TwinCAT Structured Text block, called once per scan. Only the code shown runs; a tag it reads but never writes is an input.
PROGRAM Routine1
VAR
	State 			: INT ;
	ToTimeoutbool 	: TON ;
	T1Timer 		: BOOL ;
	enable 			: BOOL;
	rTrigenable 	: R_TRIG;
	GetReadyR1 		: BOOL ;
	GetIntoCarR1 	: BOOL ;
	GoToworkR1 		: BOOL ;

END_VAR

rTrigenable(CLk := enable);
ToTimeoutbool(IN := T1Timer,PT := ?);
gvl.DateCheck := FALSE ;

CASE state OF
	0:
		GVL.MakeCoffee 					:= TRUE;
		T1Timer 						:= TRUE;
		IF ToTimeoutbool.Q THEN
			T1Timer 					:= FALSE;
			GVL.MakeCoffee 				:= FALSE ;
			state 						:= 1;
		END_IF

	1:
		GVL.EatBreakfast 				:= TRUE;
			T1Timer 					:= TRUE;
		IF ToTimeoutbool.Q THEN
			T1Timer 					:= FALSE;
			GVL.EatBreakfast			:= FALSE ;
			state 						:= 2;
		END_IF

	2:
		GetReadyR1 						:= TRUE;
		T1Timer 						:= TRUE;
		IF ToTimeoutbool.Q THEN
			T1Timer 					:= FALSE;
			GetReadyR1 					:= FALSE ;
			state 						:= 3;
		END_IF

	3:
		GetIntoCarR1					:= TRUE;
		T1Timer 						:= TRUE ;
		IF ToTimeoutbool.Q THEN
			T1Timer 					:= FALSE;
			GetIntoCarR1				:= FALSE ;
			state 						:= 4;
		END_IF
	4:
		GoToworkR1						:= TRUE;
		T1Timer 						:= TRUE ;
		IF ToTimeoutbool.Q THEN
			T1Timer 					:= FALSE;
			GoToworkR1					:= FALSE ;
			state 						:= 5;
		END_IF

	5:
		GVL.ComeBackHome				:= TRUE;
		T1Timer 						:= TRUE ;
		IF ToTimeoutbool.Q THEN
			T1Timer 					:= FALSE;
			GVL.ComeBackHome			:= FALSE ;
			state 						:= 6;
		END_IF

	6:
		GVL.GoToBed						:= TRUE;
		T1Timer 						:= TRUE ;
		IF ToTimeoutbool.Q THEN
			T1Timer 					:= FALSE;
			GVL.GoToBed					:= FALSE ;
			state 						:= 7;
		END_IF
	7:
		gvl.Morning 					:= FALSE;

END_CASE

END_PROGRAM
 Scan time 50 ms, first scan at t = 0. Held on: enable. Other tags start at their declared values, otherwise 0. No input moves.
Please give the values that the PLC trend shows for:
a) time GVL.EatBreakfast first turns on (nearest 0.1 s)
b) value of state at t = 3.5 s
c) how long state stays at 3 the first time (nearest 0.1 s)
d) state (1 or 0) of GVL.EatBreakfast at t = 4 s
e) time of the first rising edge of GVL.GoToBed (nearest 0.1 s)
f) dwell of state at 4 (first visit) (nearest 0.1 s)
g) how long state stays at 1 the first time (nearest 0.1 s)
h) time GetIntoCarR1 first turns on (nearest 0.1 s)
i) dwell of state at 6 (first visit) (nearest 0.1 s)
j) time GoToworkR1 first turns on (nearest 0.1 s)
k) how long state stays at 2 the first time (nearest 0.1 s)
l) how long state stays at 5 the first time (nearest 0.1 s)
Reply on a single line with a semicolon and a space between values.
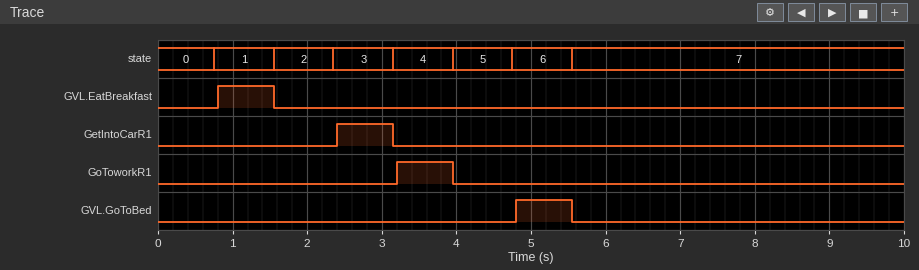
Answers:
0.8 s; 4; 0.8 s; 0; 4.8 s; 0.8 s; 0.8 s; 2.4 s; 0.8 s; 3.2 s; 0.8 s; 0.8 s
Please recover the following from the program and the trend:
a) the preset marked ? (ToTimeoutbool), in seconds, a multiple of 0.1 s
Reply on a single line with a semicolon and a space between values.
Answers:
0.7 s
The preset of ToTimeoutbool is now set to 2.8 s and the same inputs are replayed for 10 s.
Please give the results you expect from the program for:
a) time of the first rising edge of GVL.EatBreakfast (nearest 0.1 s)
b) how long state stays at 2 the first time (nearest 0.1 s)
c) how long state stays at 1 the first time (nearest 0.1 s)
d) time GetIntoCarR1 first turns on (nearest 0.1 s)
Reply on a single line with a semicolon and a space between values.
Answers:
2.9 s; 2.9 s; 2.9 s; 8.7 s
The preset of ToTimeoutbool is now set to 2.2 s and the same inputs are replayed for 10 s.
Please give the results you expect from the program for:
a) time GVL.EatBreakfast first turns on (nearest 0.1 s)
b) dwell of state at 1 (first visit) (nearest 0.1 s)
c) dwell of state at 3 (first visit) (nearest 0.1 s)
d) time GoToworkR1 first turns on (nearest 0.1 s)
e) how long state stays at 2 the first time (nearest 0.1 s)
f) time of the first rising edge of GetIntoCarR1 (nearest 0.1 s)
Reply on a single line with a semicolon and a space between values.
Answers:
2.3 s; 2.3 s; 2.3 s; 9.2 s; 2.3 s; 6.9 s
